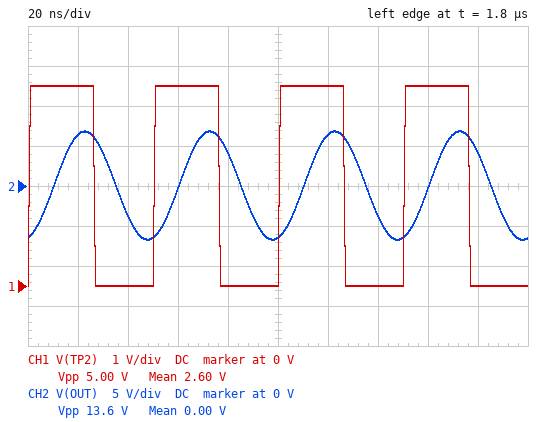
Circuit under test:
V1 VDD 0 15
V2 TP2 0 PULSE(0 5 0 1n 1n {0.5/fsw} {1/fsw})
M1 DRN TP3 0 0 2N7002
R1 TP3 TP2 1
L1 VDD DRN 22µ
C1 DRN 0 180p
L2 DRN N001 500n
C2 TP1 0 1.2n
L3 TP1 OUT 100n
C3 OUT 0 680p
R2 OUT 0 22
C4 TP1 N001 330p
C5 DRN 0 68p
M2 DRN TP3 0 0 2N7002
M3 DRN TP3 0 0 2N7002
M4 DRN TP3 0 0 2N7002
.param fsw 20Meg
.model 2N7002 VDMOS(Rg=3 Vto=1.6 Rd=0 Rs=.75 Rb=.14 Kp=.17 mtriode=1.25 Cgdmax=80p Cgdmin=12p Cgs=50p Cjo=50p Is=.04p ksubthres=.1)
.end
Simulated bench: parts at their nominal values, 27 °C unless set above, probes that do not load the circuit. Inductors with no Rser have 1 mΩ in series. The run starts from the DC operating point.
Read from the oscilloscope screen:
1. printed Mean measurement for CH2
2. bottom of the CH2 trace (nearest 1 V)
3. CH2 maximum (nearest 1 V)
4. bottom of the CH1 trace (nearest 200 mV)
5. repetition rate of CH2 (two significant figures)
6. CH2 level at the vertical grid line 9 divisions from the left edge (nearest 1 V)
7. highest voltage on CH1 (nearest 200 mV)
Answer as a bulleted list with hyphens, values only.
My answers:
- 0.00 V
- -7 V
- 7 V
- 0 V
- 20 MHz
- 4 V
- 5.0 V
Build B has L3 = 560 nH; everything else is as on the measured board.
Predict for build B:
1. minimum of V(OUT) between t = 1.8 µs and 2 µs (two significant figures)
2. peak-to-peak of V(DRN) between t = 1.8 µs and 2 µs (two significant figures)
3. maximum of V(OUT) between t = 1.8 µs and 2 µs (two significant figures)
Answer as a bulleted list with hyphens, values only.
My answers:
- -860 mV
- 42 V
- 870 mV
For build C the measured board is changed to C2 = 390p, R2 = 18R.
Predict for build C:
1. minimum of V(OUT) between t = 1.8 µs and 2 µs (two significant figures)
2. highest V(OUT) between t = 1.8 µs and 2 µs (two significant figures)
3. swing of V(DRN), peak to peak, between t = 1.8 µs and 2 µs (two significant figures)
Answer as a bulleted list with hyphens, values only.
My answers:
- -5.6 V
- 6.2 V
- 43 V
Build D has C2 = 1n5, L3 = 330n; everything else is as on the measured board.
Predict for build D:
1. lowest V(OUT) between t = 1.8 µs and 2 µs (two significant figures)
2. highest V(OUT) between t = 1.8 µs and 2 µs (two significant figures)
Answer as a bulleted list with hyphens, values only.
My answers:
- -1.3 V
- 1.3 V
